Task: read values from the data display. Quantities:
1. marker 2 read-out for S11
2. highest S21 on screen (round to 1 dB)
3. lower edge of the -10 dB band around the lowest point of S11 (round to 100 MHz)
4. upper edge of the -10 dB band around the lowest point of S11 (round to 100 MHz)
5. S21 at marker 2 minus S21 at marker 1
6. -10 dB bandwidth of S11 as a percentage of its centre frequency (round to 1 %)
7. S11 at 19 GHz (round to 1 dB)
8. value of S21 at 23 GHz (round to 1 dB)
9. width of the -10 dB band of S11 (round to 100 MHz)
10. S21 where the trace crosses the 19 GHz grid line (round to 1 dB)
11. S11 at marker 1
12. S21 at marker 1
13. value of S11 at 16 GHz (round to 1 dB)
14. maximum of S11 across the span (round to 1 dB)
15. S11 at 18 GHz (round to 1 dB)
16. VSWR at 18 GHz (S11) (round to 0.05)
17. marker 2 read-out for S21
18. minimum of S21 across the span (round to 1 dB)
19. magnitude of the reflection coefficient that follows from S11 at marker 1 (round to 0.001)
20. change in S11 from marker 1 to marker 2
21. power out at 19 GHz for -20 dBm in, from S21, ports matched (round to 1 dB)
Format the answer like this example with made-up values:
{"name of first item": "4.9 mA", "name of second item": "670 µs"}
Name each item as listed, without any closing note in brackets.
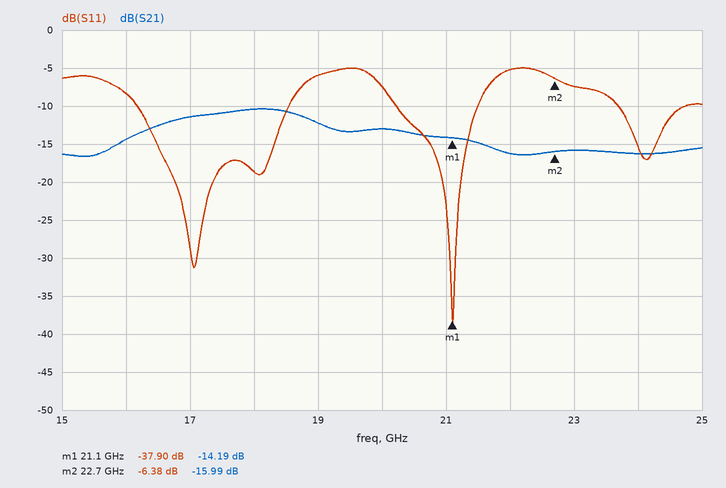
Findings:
{"marker 2 read-out for S11": "-6.38 dB", "highest S21 on screen": "-10 dB", "lower edge of the -10 dB band around the lowest point of S11": "20.2 GHz", "upper edge of the -10 dB band around the lowest point of S11": "21.5 GHz", "S21 at marker 2 minus S21 at marker 1": "-1.80 dB", "-10 dB bandwidth of S11 as a percentage of its centre frequency": "6 %", "S11 at 19 GHz": "-6 dB", "value of S21 at 23 GHz": "-16 dB", "width of the -10 dB band of S11": "1.3 GHz", "S21 where the trace crosses the 19 GHz grid line": "-12 dB", "S11 at marker 1": "-37.90 dB", "S21 at marker 1": "-14.19 dB", "value of S11 at 16 GHz": "-8 dB", "maximum of S11 across the span": "-5 dB", "S11 at 18 GHz": "-19 dB", "VSWR at 18 GHz (S11)": "1.25", "marker 2 read-out for S21": "-15.99 dB", "minimum of S21 across the span": "-17 dB", "magnitude of the reflection coefficient that follows from S11 at marker 1": "0.013", "change in S11 from marker 1 to marker 2": "31.52 dB", "power out at 19 GHz for -20 dBm in, from S21, ports matched": "-32 dBm"}
